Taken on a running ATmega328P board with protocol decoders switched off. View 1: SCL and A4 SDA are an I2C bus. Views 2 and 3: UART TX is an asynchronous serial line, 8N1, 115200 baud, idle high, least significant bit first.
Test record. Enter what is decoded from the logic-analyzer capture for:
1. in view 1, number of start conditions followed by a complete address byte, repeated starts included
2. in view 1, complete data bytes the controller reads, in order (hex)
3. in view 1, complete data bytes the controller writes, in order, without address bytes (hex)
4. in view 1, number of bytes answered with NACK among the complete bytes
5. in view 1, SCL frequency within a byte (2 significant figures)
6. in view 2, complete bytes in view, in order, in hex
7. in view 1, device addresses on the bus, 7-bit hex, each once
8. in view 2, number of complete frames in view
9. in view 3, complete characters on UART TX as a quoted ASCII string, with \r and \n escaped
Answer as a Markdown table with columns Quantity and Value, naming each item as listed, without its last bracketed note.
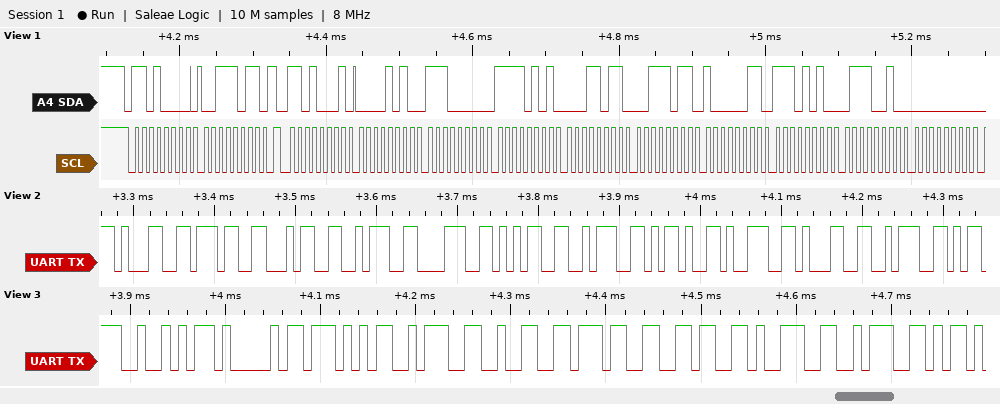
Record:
| Quantity | Value |
|---|---|
| in view 1, number of start conditions followed by a complete address byte, repeated starts included | 2 |
| in view 1, complete data bytes the controller reads, in order | 0A E0 F5 1B 3B 83 EA 72 00 |
| in view 1, complete data bytes the controller writes, in order, without address bytes | 3B |
| in view 1, number of bytes answered with NACK among the complete bytes | 0 |
| in view 1, SCL frequency within a byte | 100 kHz |
| in view 2, complete bytes in view, in order, in hex | 31 37 34 3A 38 35 3A 2D 39 31 3A |
| in view 1, device addresses on the bus, 7-bit hex, each once | 0x68 |
| in view 2, number of complete frames in view | 11 |
| in view 3, complete characters on UART TX as a quoted ASCII string, with \r and \n escaped | "RAW:2769:" |
